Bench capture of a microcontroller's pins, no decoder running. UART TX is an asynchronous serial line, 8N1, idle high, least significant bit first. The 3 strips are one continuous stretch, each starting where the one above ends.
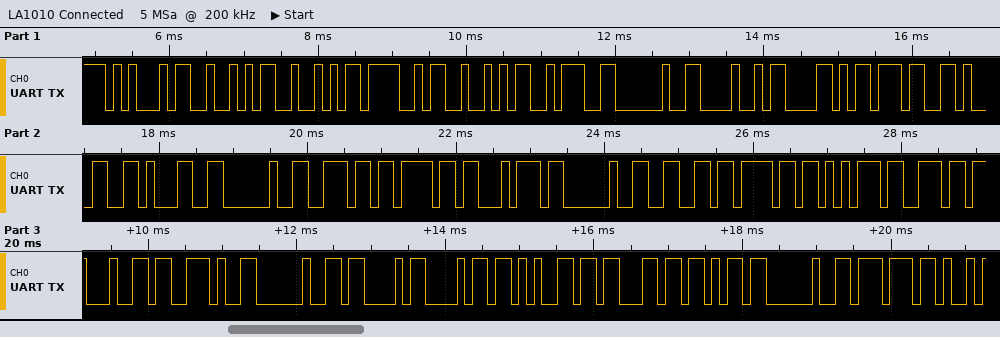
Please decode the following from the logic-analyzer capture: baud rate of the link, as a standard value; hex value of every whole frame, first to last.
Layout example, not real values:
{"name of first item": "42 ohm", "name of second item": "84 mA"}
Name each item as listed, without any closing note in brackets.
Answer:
{"baud rate of the link, as a standard value": "9600 baud", "hex value of every whole frame, first to last": "0x45 0x52 0x52 0x4F 0x52 0x3A 0x20 0x48 0x58 0x37 0x31 0x31 0x20 0x6E 0x6F 0x74 0x20 0x66 0x6F 0x75 0x6E 0x64 0x2E 0x20 0x43 0x68 0x65 0x63 0x6B 0x20 0x77"}
